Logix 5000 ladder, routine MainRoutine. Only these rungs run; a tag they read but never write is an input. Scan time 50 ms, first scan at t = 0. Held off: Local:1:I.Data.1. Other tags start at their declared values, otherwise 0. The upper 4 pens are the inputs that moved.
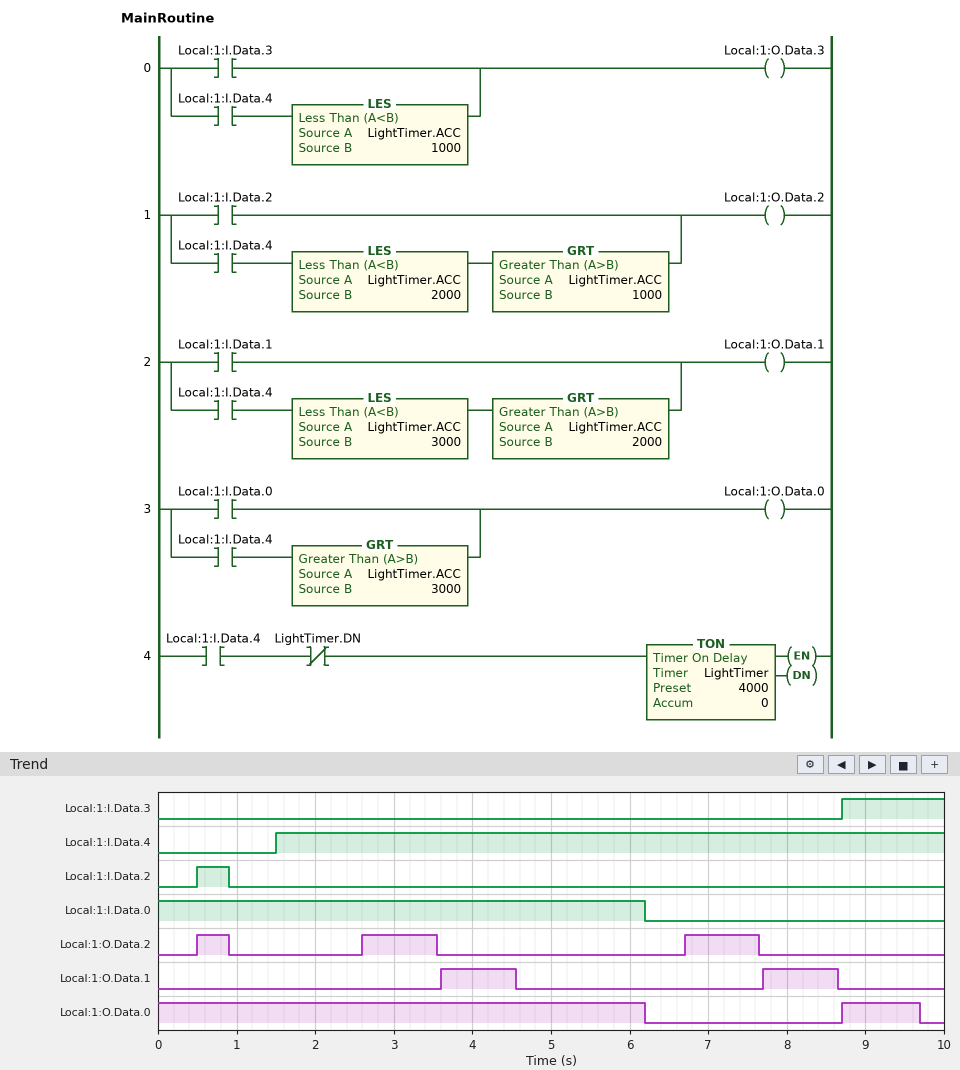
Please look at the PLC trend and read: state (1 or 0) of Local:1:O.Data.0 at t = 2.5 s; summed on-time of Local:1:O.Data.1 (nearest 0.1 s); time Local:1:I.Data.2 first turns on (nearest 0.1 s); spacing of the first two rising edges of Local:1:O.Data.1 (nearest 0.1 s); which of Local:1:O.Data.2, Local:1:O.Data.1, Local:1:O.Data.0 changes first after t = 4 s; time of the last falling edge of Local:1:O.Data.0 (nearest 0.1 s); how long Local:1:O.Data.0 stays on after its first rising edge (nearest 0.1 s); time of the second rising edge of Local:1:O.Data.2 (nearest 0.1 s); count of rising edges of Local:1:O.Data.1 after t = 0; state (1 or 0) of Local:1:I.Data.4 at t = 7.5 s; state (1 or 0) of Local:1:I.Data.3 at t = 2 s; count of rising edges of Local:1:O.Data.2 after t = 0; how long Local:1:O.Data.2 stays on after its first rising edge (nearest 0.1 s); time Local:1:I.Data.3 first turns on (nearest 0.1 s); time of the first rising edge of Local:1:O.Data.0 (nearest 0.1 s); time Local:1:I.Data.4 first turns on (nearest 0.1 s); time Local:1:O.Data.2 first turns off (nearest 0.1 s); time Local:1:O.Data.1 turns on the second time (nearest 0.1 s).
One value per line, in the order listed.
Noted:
1
1.9 s
0.5 s
4.1 s
Local:1:O.Data.1
9.7 s
1.0 s
2.6 s
2
1
0
3
0.4 s
8.7 s
8.7 s
1.5 s
0.9 s
7.7 s
